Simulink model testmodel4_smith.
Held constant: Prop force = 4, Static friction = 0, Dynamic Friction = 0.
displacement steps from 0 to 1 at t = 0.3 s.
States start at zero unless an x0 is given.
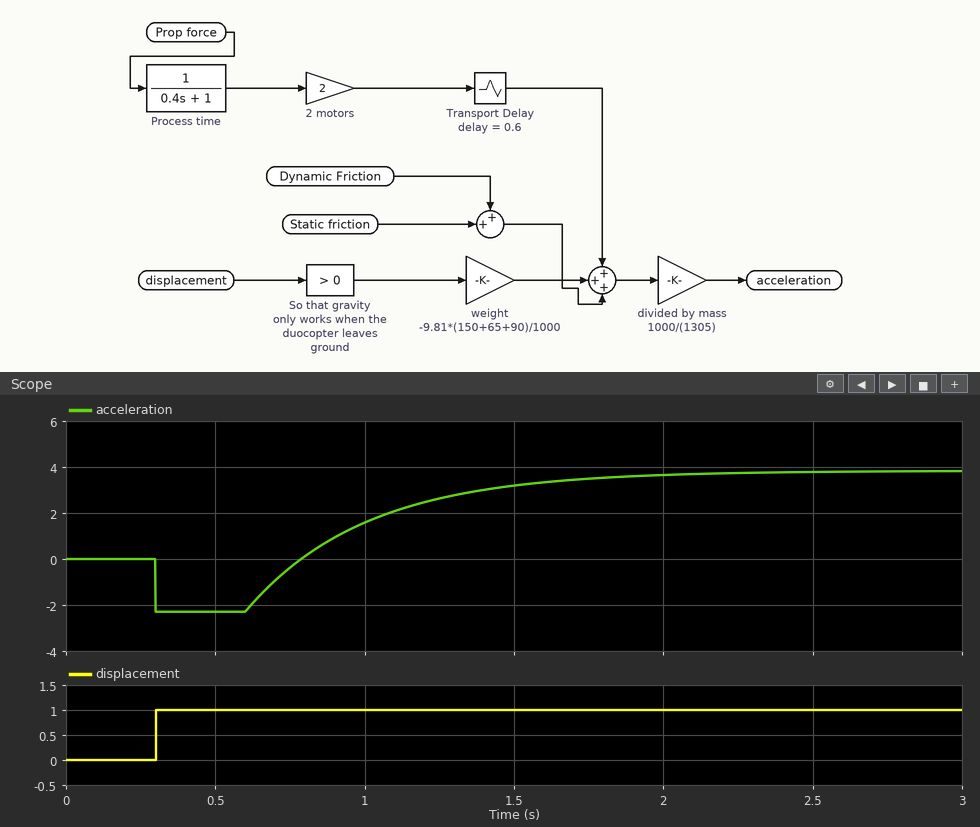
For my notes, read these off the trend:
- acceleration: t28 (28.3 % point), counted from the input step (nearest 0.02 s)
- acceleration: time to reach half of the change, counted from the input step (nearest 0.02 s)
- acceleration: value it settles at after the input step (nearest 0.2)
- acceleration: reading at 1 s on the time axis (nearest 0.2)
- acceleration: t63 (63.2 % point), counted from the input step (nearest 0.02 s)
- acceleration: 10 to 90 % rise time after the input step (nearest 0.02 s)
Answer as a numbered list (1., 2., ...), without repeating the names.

1. 0.62 s
2. 0.76 s
3. 3.8
4. 1.6
5. 0.88 s
6. 0.88 s
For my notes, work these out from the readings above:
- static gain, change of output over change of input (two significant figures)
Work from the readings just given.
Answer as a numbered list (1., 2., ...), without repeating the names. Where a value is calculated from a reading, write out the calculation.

1. (3.8 - 0) / (1 - 0) = 3.8
